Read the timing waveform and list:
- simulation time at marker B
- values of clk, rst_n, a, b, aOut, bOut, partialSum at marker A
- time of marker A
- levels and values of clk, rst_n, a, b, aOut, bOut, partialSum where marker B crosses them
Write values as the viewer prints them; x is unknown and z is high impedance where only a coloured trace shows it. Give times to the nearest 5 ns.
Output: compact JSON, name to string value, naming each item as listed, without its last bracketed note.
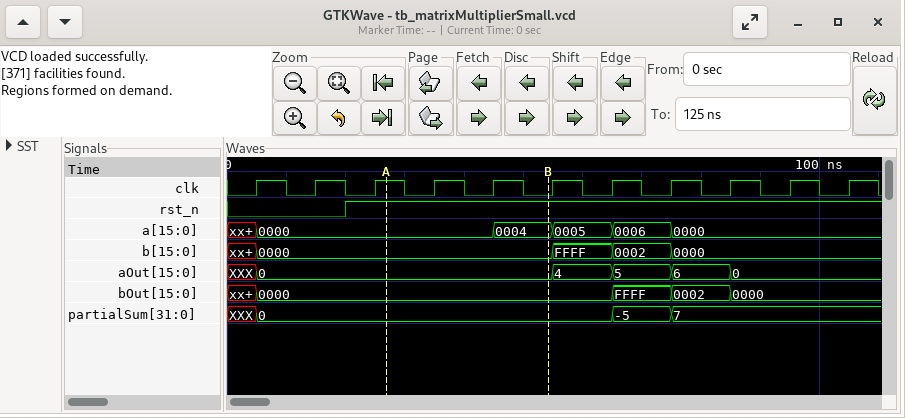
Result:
{"simulation time at marker B": "55 ns", "values of clk, rst_n, a, b, aOut, bOut, partialSum at marker A": "clk=1, rst_n=1, a=0000, b=0000, aOut=0, bOut=0000, partialSum=0", "time of marker A": "25 ns", "levels and values of clk, rst_n, a, b, aOut, bOut, partialSum where marker B crosses them": "clk=0, rst_n=1, a=0004, b=0000, aOut=0, bOut=0000, partialSum=0"}
